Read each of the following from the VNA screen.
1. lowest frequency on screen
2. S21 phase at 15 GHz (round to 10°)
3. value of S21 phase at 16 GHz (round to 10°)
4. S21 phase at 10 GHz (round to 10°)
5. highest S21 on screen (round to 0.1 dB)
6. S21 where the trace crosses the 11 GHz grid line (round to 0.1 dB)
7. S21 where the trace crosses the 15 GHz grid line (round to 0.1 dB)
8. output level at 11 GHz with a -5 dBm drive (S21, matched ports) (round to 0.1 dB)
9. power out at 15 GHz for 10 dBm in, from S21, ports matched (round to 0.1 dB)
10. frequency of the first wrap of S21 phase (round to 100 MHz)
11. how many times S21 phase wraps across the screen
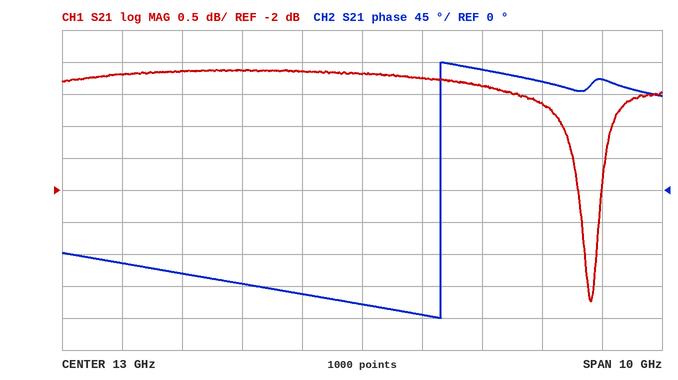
8 GHz
170°
150°
-120°
-0.1 dB
-0.1 dB
-0.4 dB
-5.1 dBm
9.6 dBm
14.3 GHz
1
